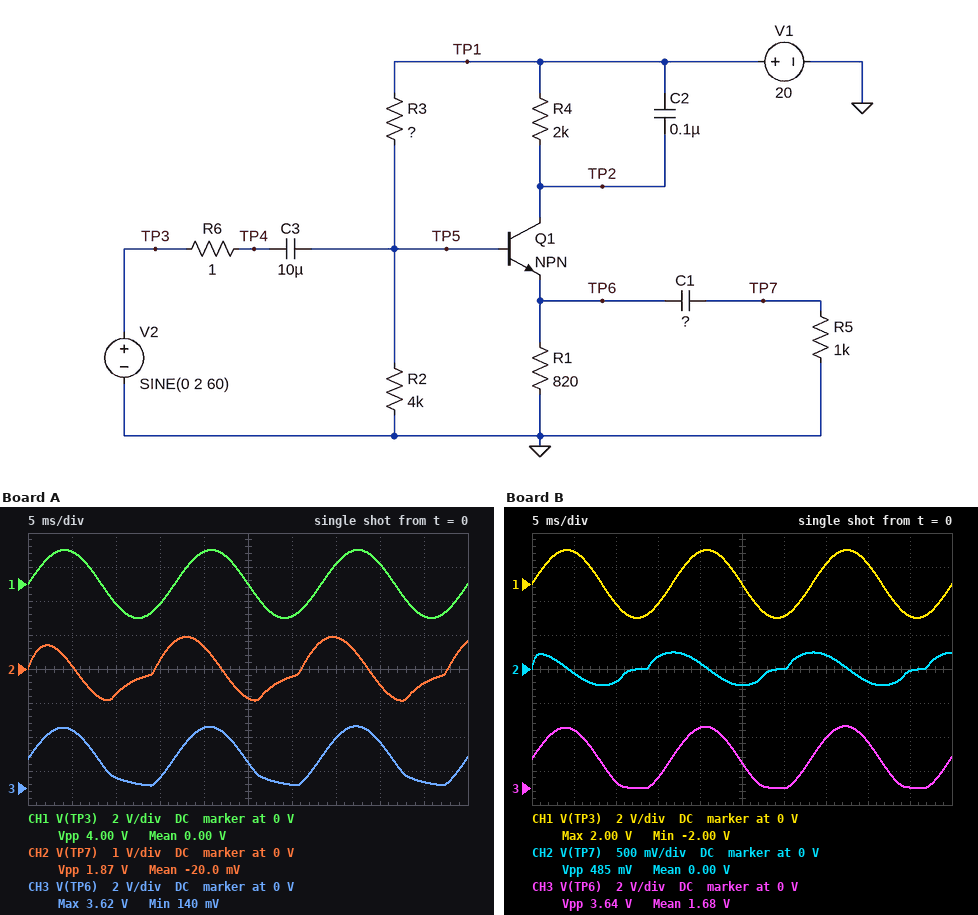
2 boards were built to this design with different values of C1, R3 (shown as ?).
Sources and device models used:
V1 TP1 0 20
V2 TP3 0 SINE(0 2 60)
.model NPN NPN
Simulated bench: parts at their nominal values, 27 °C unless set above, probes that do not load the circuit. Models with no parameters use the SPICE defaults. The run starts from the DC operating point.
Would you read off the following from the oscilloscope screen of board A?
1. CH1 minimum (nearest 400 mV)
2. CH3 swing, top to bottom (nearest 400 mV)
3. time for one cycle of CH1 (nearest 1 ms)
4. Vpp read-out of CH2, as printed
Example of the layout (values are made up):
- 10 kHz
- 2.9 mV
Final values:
- -2.0 V
- 3.6 V
- 17 ms
- 1.87 V
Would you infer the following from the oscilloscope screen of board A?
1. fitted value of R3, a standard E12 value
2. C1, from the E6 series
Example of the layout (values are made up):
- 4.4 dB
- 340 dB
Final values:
- 27 kΩ
- 1.5 µF
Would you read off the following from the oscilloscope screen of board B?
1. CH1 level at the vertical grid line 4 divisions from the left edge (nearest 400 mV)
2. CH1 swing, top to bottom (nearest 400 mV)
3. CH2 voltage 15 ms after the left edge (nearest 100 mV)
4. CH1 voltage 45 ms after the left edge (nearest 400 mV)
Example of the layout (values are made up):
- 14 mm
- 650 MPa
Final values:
- 2.0 V
- 4.0 V
- 200 mV
- -2.0 V
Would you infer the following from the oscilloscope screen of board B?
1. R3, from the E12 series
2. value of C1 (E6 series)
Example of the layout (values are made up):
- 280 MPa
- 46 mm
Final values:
- 27 kΩ
- 330 nF
